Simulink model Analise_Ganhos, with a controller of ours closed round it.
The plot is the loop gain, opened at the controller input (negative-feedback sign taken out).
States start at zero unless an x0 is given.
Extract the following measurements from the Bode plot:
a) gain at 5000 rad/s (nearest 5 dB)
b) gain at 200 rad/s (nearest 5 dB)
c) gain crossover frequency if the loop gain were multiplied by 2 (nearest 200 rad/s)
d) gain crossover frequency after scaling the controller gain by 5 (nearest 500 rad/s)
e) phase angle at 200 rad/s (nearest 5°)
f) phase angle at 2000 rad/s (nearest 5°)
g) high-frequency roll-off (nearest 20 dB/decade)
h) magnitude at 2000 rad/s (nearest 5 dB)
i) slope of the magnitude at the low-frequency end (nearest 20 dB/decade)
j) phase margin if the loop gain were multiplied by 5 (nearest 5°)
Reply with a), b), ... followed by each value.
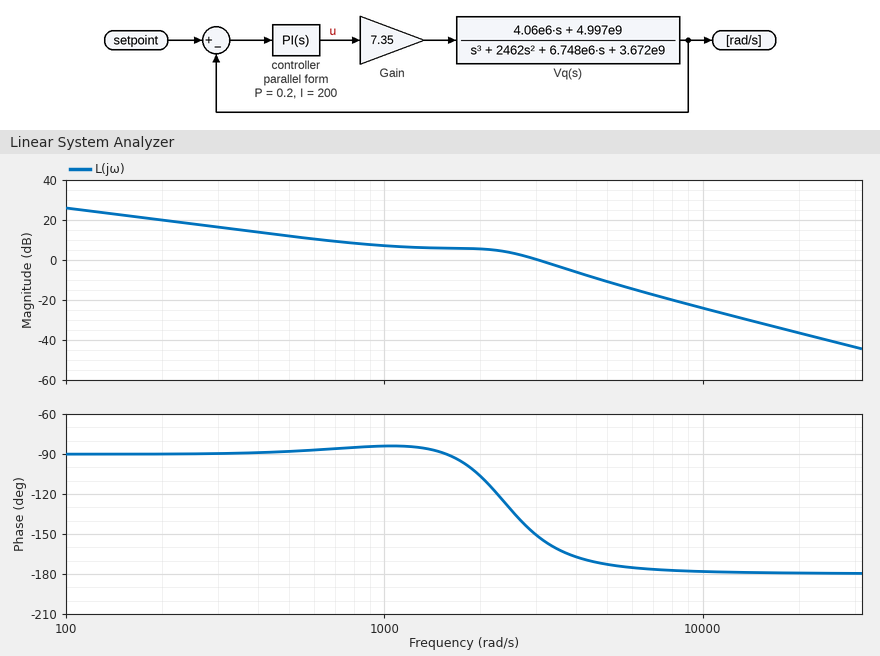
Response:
a) -10 dB
b) 20 dB
c) 4000 rad/s
d) 6000 rad/s
e) -90°
f) -105°
g) -40 dB/decade
h) 5 dB
i) -20 dB/decade
j) 5°
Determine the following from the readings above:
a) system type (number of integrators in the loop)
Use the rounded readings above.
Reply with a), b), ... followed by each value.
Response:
a) 1
